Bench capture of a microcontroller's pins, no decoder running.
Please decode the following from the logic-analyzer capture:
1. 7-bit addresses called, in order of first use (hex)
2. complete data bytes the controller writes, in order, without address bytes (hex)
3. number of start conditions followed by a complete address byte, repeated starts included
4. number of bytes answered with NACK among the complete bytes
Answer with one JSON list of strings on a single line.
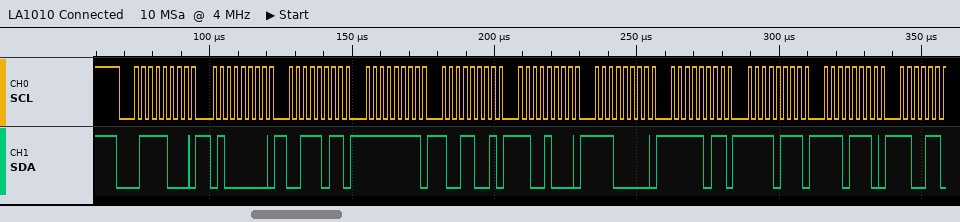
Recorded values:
["0x3C", "40 3B FF 99 C8 E0 FB F7 EE", "1", "0"]
